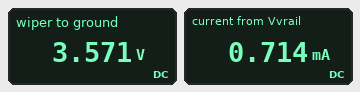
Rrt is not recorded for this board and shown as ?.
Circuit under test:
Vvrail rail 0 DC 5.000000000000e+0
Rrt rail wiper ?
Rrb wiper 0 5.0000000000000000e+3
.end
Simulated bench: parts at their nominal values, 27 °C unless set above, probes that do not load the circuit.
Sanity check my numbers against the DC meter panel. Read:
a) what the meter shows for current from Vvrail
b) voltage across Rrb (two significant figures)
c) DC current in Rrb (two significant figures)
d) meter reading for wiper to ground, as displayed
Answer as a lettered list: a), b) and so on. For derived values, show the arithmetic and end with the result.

a) 0.714 mA
b) 3.571 V = 3.6 V
c) (3.571 V) / 5 kΩ = 710 µA
d) 3.571 V
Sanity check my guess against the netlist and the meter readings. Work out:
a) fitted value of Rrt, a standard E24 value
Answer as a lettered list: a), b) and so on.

a) 2 kΩ
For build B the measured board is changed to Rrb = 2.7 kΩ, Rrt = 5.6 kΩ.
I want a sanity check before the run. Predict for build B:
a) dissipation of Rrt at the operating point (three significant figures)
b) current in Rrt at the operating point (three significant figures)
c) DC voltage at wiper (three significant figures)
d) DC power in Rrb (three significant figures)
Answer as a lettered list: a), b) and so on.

a) 2.03 mW
b) 602 µA
c) 1.63 V
d) 980 µW
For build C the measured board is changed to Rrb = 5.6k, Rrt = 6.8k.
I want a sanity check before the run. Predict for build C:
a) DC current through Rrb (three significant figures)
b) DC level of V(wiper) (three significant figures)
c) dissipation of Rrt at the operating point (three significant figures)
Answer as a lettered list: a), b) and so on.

a) 403 µA
b) 2.26 V
c) 1.11 mW
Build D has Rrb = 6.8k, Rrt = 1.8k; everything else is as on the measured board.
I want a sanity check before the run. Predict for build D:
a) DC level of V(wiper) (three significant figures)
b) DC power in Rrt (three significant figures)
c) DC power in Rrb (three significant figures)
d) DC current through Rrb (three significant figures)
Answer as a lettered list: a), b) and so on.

a) 3.95 V
b) 608 µW
c) 2.30 mW
d) 581 µA
